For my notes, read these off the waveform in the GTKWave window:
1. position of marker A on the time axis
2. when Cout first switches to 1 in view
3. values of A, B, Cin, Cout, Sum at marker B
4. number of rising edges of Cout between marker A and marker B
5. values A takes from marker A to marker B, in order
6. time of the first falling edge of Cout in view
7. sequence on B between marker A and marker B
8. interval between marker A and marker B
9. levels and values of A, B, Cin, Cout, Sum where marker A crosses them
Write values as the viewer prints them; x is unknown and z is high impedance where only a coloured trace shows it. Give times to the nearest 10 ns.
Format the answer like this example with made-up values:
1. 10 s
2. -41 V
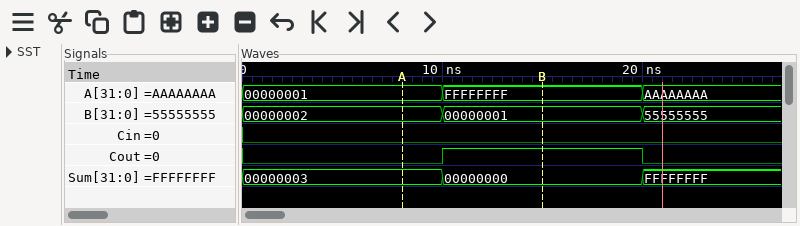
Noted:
1. 10 ns
2. 10 ns
3. A=FFFFFFFF, B=00000001, Cin=0, Cout=1, Sum=00000000
4. 1
5. 00000001, FFFFFFFF
6. 20 ns
7. 00000002, 00000001
8. 10 ns
9. A=00000001, B=00000002, Cin=0, Cout=0, Sum=00000003
